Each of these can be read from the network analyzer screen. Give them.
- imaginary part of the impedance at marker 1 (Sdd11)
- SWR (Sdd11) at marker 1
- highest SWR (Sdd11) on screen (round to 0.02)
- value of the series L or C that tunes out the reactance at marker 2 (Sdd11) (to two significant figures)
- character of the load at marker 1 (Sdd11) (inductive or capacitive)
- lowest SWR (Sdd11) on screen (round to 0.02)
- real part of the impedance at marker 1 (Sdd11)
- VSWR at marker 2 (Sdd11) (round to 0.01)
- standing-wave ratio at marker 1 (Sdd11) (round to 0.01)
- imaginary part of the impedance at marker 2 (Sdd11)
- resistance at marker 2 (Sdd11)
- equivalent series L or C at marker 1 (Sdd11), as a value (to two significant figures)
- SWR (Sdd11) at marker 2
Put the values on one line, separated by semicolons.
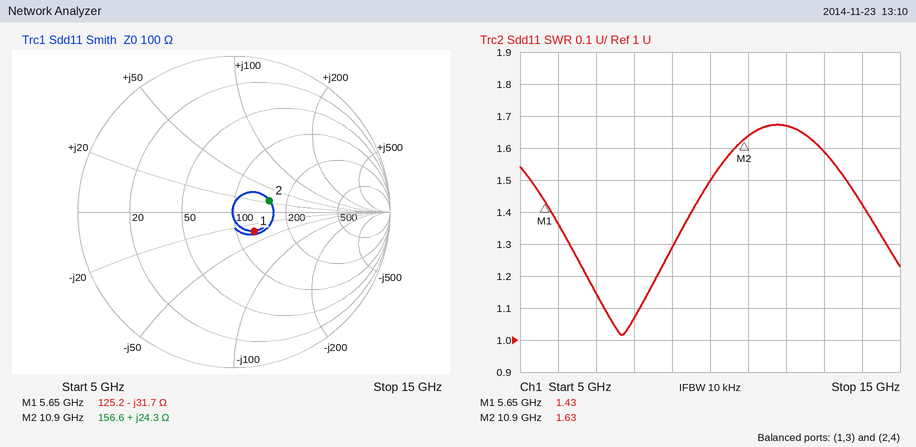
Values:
-31.7 Ω; 1.43; 1.68; 600 fF; capacitive; 1.02; 125.2 Ω; 1.63; 1.43; +24.3 Ω; 156.6 Ω; 890 fF; 1.63
